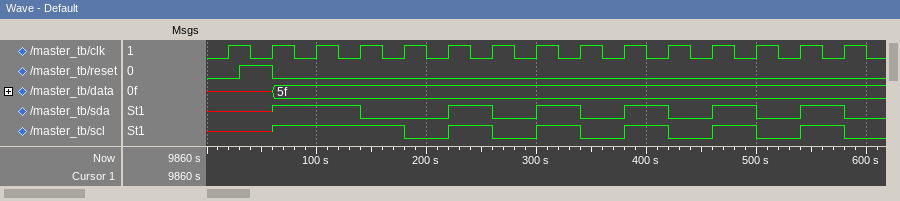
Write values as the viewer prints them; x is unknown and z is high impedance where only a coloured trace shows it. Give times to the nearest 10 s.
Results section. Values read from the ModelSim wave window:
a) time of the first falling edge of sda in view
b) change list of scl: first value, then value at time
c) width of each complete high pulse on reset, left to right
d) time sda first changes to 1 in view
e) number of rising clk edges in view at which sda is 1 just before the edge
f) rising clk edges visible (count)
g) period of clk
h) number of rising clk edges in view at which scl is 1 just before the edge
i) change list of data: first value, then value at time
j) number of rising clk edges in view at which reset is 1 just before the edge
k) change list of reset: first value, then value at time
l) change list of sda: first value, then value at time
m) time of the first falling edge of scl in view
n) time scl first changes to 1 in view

140 s
x, 1 at 60 s, 0 at 180 s, 1 at 220 s, 0 at 260 s, 1 at 300 s, 0 at 340 s, 1 at 380 s, 0 at 420 s, 1 at 460 s, 0 at 500 s, 1 at 540 s, 0 at 580 s
30 s
60 s
7
15
40 s
8
x, 5f at 60 s
1
0, 1 at 30 s, 0 at 60 s
x, 1 at 60 s, 0 at 140 s, 1 at 220 s, 0 at 260 s, 1 at 300 s, 0 at 340 s, 1 at 380 s, 0 at 420 s, 1 at 460 s, 0 at 500 s, 1 at 540 s, 0 at 580 s
180 s
60 s
